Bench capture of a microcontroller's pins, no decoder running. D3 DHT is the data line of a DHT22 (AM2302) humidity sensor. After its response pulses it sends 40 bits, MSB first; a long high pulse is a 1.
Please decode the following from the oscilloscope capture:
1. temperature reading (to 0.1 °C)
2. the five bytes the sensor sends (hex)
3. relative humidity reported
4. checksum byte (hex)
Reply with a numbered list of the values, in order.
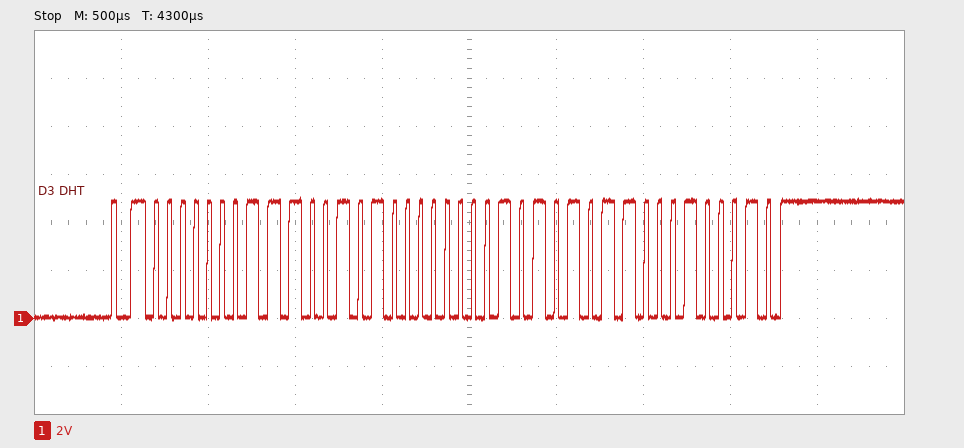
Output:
1. 34.2 °C
2. 01 CA 01 56 22
3. 45.8 %
4. 0x22
